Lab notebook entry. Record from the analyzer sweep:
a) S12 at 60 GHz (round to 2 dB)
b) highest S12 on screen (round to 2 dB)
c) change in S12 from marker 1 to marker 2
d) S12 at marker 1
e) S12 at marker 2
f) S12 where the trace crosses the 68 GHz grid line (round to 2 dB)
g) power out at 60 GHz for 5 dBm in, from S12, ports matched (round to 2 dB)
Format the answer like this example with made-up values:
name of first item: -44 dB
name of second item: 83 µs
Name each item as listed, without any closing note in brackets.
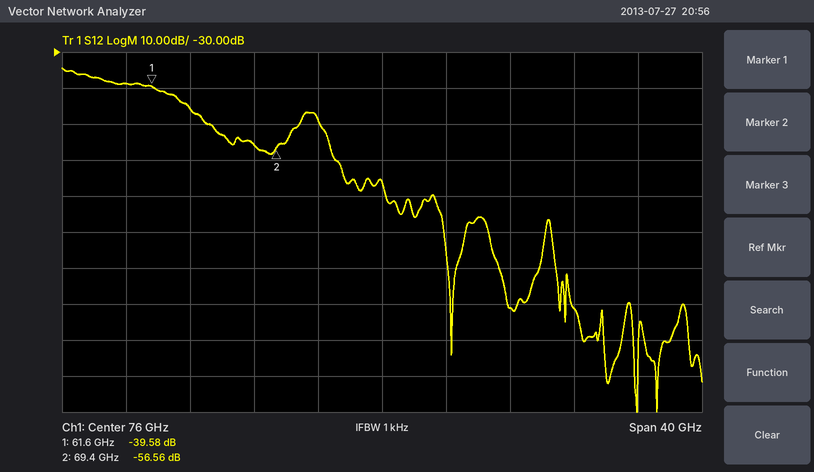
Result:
S12 at 60 GHz: -38 dB
highest S12 on screen: -34 dB
change in S12 from marker 1 to marker 2: -16.98 dB
S12 at marker 1: -39.58 dB
S12 at marker 2: -56.56 dB
S12 where the trace crosses the 68 GHz grid line: -56 dB
power out at 60 GHz for 5 dBm in, from S12, ports matched: -34 dBm
